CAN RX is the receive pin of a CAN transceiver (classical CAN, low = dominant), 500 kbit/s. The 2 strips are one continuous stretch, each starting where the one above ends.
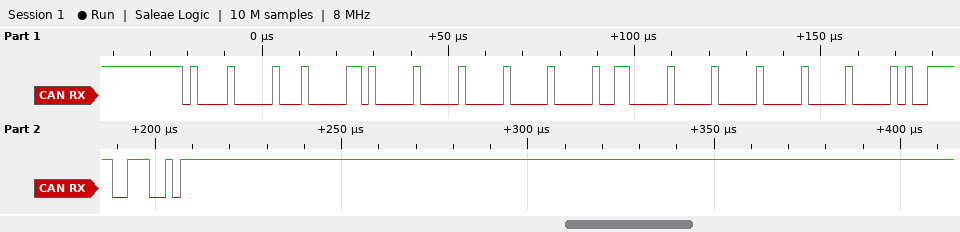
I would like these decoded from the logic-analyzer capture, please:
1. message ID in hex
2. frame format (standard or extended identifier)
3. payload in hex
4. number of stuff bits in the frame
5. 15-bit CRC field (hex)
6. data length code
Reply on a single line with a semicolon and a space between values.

0x420; standard; 28 00 00 00 C0 00 00 00; 14; 0x27DC; 8
